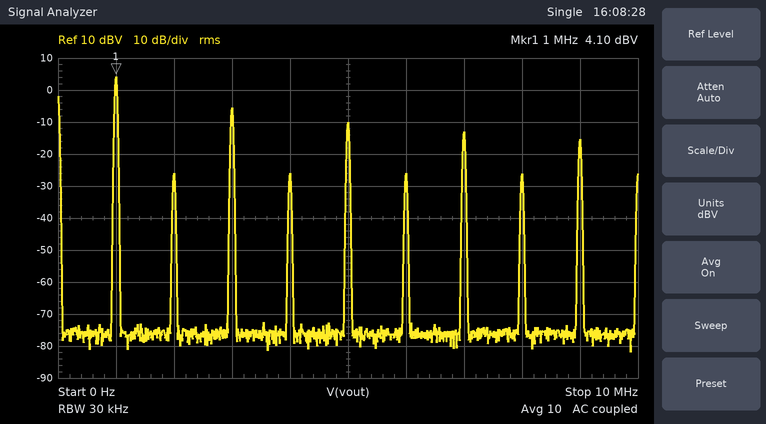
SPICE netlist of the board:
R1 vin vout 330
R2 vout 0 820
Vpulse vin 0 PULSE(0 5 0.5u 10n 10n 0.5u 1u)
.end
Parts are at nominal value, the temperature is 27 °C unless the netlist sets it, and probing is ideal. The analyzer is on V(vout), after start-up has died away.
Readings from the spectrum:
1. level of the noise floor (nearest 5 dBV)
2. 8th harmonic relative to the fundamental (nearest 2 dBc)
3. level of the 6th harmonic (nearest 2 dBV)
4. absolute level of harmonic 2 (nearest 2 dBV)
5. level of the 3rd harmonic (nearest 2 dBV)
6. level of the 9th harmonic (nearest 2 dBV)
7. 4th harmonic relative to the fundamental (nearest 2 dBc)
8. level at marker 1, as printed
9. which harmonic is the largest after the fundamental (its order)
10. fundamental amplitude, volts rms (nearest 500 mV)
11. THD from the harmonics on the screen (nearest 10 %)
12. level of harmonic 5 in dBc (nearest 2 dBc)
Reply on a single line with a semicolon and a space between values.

-75 dBV; -30 dBc; -26 dBV; -26 dBV; -6 dBV; -16 dBV; -30 dBc; 4.10 dBV; 3; 1.5 V; 40 %; -14 dBc
